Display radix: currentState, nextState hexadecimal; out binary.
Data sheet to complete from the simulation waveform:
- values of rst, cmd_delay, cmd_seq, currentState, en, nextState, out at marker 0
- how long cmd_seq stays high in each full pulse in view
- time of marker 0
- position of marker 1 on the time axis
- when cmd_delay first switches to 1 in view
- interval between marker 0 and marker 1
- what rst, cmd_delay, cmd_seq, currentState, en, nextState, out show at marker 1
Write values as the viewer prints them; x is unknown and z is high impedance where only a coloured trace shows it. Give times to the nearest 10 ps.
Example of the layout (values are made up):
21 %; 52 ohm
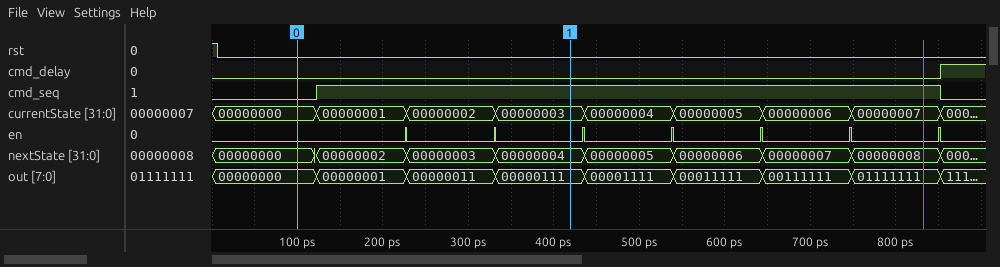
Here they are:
rst=0, cmd_delay=0, cmd_seq=0, currentState=00000000, en=0, nextState=00000000, out=00000000; 730 ps; 100 ps; 420 ps; 850 ps; 320 ps; rst=0, cmd_delay=0, cmd_seq=1, currentState=00000003, en=0, nextState=00000004, out=00000111
